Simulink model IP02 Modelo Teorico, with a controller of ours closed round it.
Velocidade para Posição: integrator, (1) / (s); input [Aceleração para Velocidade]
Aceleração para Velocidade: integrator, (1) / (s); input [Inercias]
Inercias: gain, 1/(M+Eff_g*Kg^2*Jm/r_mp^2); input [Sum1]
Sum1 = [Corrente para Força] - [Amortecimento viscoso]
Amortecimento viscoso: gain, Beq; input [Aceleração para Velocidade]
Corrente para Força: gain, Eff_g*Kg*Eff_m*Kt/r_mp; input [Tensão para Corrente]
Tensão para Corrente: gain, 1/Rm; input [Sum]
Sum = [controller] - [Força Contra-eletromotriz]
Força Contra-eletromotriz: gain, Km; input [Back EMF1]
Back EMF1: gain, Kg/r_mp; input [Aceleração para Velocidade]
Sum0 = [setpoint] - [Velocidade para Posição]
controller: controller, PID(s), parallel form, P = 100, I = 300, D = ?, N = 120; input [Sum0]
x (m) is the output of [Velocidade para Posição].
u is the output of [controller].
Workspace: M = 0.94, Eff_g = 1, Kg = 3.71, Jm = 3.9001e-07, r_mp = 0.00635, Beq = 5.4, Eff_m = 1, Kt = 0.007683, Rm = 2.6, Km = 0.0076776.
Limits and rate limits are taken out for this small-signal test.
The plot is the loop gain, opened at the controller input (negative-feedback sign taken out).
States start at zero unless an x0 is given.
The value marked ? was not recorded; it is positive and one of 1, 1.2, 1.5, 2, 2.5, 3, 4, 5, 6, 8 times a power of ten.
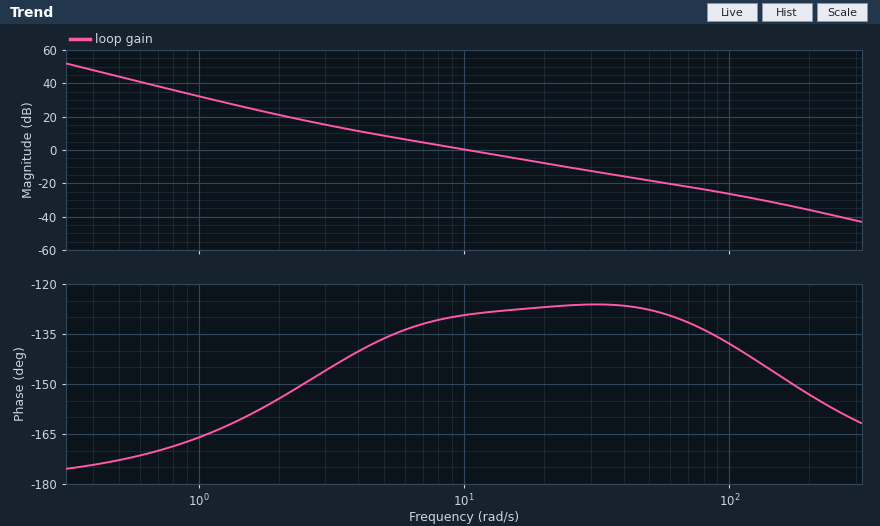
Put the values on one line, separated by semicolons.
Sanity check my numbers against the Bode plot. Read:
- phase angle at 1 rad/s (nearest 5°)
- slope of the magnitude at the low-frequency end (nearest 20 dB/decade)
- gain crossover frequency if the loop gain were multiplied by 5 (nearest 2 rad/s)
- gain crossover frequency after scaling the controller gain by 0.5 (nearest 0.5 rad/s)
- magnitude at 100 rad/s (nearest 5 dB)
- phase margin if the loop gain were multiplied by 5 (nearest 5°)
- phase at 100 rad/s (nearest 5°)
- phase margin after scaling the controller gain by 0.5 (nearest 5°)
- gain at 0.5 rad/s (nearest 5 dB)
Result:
-165°; -40 dB/decade; 34 rad/s; 6.0 rad/s; -25 dB; 55°; -140°; 45°; 45 dB
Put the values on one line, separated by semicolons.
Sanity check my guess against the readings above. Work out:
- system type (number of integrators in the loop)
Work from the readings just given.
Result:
2
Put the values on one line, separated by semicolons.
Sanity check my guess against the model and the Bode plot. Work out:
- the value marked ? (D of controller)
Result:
3
